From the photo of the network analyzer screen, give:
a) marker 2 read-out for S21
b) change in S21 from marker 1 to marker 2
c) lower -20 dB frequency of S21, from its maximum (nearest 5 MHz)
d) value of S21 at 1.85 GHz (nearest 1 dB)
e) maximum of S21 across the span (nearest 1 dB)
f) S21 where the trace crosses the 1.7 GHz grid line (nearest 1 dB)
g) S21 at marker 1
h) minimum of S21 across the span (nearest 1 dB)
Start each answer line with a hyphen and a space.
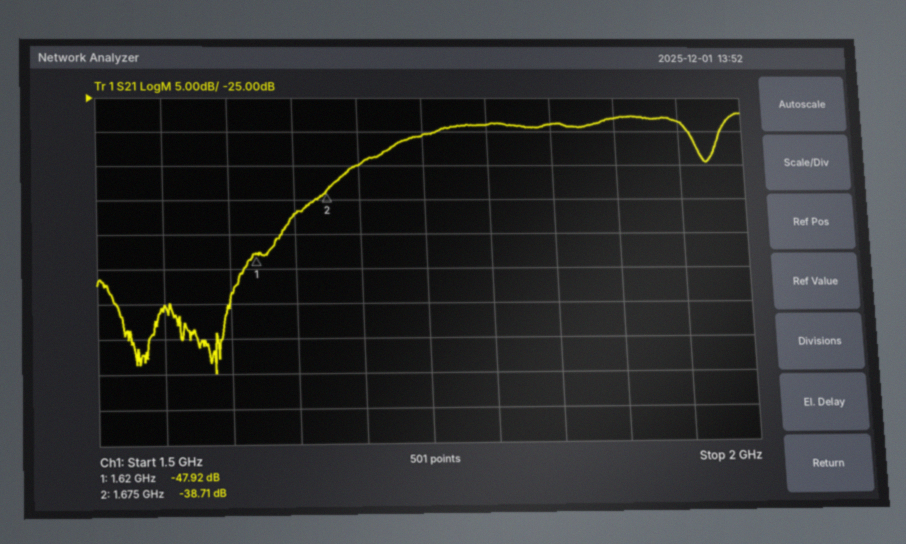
- -38.71 dB
- 9.21 dB
- 1.630 GHz
- -29 dB
- -27 dB
- -35 dB
- -47.92 dB
- -65 dB
